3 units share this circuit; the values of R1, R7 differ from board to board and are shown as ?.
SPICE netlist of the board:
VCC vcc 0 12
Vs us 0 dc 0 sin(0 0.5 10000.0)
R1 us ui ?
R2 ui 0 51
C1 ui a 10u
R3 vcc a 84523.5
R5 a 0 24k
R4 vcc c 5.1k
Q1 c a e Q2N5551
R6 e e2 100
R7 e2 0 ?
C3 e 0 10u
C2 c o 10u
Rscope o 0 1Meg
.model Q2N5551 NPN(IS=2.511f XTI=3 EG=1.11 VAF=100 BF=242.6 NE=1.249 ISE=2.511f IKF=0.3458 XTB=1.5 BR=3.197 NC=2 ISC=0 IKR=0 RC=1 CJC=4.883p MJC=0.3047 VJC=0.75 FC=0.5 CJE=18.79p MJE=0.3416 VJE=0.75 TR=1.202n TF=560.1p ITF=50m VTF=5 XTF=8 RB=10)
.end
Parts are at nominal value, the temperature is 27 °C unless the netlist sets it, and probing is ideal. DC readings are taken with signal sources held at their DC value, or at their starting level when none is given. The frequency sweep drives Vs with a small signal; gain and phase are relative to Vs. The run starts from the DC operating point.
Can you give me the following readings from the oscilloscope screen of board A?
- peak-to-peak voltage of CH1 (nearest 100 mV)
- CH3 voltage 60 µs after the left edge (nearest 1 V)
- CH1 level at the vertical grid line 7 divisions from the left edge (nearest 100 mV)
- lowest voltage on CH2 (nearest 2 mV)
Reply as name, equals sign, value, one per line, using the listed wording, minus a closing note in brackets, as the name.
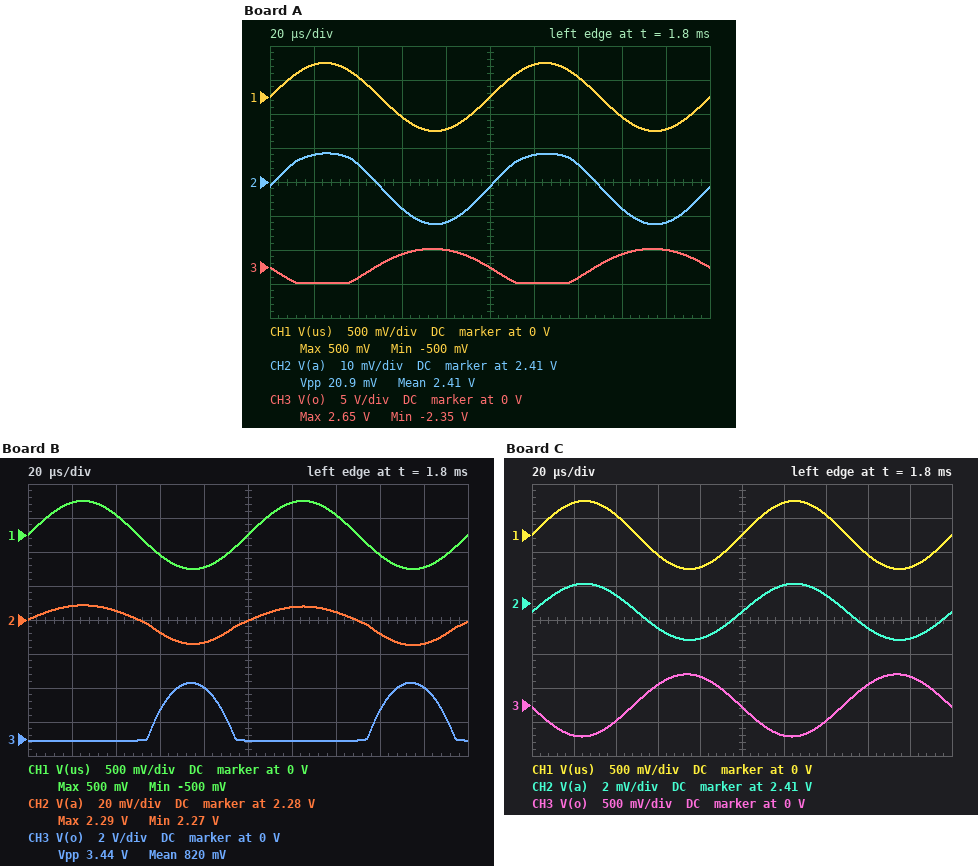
peak-to-peak voltage of CH1 = 1.0 V
CH3 voltage 60 µs after the left edge = 2 V
CH1 level at the vertical grid line 7 divisions from the left edge = 300 mV
lowest voltage on CH2 = 2.398 V
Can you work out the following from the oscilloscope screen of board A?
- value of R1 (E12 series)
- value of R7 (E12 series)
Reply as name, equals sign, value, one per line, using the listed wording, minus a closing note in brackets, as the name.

value of R1 = 2.2 kΩ
value of R7 = 1 kΩ
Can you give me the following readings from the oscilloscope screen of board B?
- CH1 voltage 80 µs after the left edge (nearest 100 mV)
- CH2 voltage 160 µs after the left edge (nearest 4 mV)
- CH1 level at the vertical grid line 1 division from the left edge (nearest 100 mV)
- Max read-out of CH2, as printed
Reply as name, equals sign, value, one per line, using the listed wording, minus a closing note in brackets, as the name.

CH1 voltage 80 µs after the left edge = -500 mV
CH2 voltage 160 µs after the left edge = 2.272 V
CH1 level at the vertical grid line 1 division from the left edge = 500 mV
Max read-out of CH2, as printed = 2.29 V
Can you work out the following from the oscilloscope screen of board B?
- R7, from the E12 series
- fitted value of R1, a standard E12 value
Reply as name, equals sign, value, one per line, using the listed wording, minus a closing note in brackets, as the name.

R7, from the E12 series = 680 Ω
fitted value of R1, a standard E12 value = 1.5 kΩ
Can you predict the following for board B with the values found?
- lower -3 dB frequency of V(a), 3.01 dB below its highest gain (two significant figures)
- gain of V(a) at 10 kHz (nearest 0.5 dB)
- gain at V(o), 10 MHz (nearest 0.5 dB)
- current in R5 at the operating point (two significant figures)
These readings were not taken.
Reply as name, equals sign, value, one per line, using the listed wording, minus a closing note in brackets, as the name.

lower -3 dB frequency of V(a), 3.01 dB below its highest gain = 5.9 Hz
gain of V(a) at 10 kHz = -33.5 dB
gain at V(o), 10 MHz = -1.0 dB
current in R5 at the operating point = 96 µA
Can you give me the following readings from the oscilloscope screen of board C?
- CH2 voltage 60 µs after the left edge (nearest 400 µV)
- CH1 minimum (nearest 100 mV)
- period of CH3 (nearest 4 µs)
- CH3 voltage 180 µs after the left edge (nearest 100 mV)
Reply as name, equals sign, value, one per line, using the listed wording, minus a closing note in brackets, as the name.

CH2 voltage 60 µs after the left edge = 2.4084 V
CH1 minimum = -500 mV
period of CH3 = 100 µs
CH3 voltage 180 µs after the left edge = 400 mV
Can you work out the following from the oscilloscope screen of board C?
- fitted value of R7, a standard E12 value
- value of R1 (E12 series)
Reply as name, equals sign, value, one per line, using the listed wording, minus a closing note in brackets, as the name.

fitted value of R7, a standard E12 value = 1 kΩ
value of R1 = 15 kΩ
